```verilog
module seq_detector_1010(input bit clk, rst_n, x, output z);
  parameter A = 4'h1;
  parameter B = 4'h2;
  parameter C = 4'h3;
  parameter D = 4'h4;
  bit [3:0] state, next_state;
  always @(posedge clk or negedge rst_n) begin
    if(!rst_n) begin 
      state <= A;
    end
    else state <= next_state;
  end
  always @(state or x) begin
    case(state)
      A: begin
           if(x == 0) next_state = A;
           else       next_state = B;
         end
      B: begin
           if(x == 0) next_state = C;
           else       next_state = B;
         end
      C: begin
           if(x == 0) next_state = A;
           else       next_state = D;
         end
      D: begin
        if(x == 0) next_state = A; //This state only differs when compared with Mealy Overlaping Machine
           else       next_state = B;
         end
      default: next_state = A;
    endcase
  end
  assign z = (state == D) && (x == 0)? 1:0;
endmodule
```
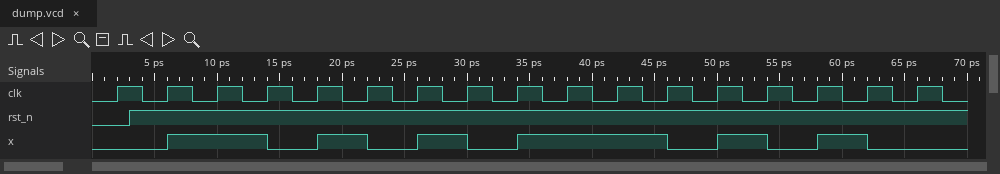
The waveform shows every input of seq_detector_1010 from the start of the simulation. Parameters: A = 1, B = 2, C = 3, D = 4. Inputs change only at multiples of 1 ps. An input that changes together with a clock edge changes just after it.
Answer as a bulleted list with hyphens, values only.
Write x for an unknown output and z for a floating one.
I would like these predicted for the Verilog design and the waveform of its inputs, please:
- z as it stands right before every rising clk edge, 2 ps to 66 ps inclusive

- 0 0 0 0 0 0 1 0 0 0 0 0 0 0 1 0 0
